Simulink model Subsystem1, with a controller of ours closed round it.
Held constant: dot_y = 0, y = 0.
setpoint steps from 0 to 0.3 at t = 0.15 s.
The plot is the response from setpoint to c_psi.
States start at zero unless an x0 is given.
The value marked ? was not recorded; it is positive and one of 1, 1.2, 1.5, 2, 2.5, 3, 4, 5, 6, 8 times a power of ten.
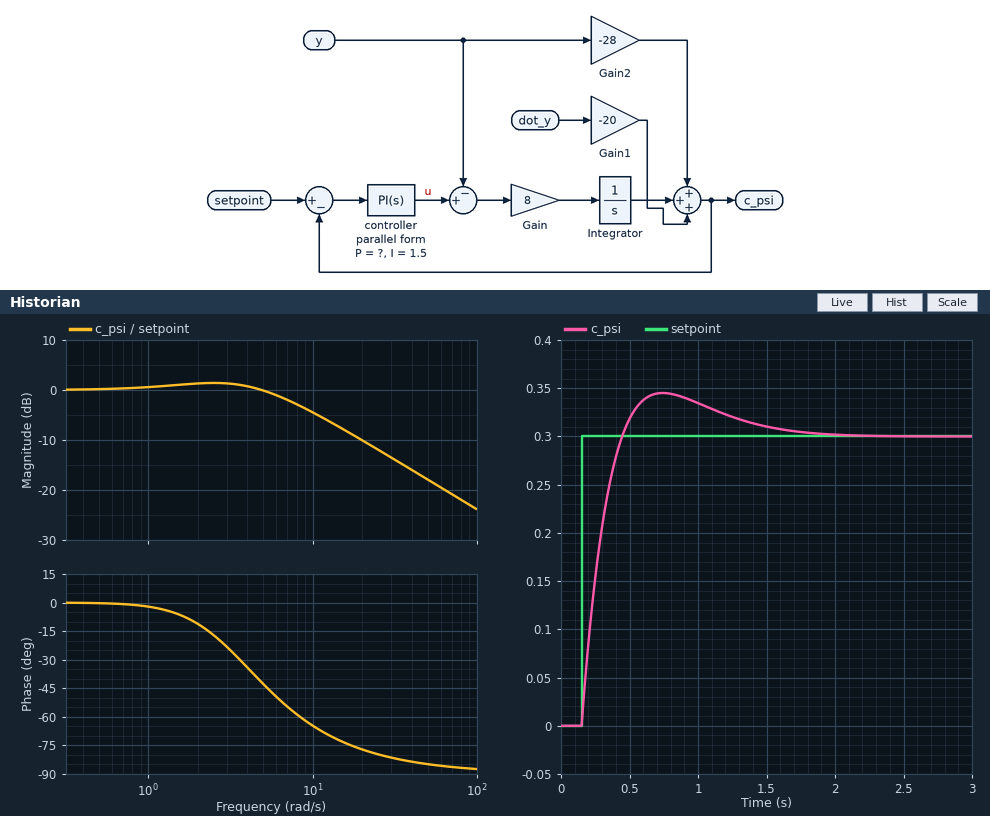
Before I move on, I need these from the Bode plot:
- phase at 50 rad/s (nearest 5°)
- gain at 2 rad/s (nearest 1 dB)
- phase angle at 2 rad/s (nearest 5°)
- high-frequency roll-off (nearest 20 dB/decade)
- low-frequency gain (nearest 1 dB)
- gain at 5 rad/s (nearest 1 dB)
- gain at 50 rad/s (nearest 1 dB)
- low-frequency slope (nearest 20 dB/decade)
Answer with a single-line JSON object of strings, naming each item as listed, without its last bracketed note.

{"phase at 50 rad/s": "-85°", "gain at 2 rad/s": "1 dB", "phase angle at 2 rad/s": "-10°", "high-frequency roll-off": "-20 dB/decade", "low-frequency gain": "0 dB", "gain at 5 rad/s": "0 dB", "gain at 50 rad/s": "-18 dB", "low-frequency slope": "0 dB/decade"}
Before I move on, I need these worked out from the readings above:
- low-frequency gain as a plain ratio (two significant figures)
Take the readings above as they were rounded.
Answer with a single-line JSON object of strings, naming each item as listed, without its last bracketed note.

{"low-frequency gain as a plain ratio": "1.0"}
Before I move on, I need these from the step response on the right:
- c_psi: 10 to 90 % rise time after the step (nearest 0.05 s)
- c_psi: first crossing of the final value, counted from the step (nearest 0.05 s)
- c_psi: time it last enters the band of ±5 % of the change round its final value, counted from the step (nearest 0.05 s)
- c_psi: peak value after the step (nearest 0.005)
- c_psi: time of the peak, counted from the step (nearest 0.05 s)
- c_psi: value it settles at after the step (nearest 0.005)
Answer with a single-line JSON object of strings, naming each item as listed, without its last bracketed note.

{"c_psi: 10 to 90 % rise time after the step": "0.20 s", "c_psi: first crossing of the final value, counted from the step": "0.30 s", "c_psi: time it last enters the band of ±5 % of the change round its final value, counted from the step": "1.20 s", "c_psi: peak value after the step": "0.345", "c_psi: time of the peak, counted from the step": "0.60 s", "c_psi: value it settles at after the step": "0.300"}
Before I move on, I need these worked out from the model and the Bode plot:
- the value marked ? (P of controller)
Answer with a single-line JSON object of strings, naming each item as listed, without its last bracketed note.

{"the value marked ?": "0.8"}
